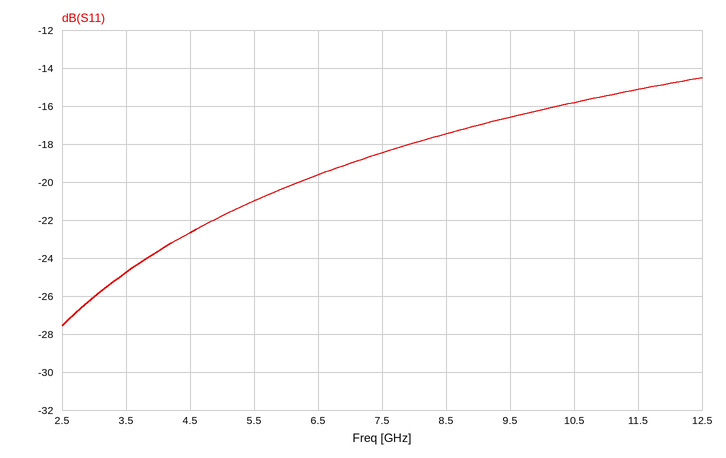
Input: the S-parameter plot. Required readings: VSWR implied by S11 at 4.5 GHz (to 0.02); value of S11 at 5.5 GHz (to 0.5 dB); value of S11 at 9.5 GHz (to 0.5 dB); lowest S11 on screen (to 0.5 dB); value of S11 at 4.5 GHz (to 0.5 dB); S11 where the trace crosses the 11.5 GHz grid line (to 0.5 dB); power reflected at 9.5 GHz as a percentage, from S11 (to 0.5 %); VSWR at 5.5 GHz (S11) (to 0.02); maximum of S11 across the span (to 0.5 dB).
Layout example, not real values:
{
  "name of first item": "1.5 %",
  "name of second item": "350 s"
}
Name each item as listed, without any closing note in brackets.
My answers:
{
  "VSWR implied by S11 at 4.5 GHz": "1.16",
  "value of S11 at 5.5 GHz": "-21.0 dB",
  "value of S11 at 9.5 GHz": "-16.5 dB",
  "lowest S11 on screen": "-27.5 dB",
  "value of S11 at 4.5 GHz": "-22.5 dB",
  "S11 where the trace crosses the 11.5 GHz grid line": "-15.0 dB",
  "power reflected at 9.5 GHz as a percentage, from S11": "2.0 %",
  "VSWR at 5.5 GHz (S11)": "1.20",
  "maximum of S11 across the span": "-14.5 dB"
}
